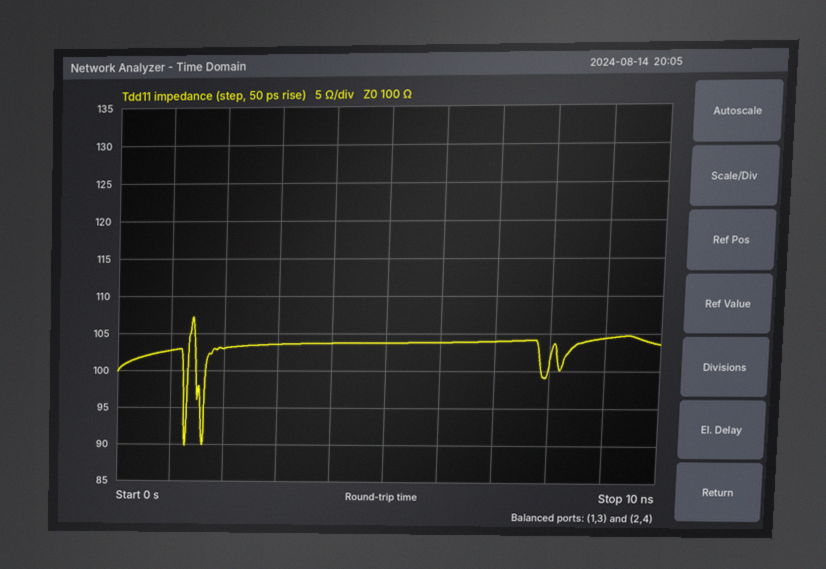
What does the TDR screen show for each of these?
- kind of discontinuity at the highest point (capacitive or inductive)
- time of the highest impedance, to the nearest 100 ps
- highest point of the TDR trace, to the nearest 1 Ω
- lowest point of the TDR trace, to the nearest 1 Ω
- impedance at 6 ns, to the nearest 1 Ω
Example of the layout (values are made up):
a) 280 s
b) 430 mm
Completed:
a) inductive
b) 1.4 ns
c) 107 Ω
d) 90 Ω
e) 104 Ω
